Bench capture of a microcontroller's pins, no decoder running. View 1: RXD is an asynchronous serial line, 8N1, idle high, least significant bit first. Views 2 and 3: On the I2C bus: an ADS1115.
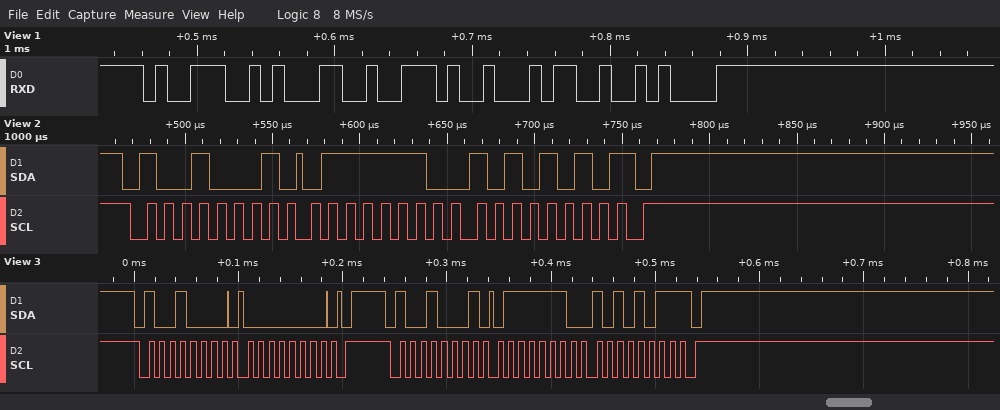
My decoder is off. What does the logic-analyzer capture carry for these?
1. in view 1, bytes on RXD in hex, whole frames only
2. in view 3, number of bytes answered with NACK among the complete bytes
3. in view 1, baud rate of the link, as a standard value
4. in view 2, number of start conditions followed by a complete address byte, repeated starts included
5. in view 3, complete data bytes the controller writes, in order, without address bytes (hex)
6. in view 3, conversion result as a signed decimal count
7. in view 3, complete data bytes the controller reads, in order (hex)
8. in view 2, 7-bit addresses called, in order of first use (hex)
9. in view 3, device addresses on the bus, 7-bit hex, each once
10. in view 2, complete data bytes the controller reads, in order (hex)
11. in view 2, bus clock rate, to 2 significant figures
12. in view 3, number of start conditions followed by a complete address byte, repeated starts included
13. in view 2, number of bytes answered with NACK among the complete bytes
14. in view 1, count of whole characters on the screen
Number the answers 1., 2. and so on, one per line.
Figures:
1. 39 31 2E 34 0A
2. 1
3. 115200 baud
4. 1
5. 00
6. 32427
7. 7E AB
8. 0x48
9. 0x48
10. 7E AA
11. 100 kHz
12. 2
13. 1
14. 5
